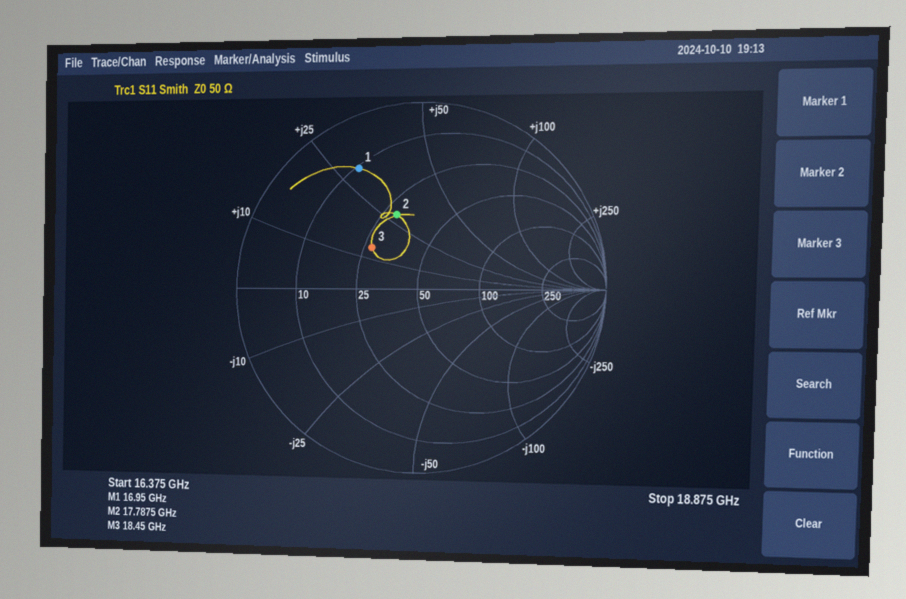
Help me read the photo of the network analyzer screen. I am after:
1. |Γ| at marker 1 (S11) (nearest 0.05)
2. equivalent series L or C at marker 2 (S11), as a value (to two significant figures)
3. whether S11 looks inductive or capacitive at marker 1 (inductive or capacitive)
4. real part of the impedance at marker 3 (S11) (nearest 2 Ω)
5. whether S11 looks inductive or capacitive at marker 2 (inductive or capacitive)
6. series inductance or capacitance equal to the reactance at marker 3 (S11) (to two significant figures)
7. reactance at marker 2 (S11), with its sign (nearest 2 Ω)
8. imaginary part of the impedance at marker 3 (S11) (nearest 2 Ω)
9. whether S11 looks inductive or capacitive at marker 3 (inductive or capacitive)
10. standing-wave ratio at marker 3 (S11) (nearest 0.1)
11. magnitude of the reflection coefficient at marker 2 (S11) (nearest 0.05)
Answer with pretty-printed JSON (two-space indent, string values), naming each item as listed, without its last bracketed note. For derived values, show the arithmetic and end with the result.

{
  "|Γ| at marker 1 (S11)": "0.75",
  "equivalent series L or C at marker 2 (S11), as a value": "L = 28 Ω/(2π × 17.7875 GHz) ≈ 251 pH, so 250 pH to two significant figures",
  "whether S11 looks inductive or capacitive at marker 1": "inductive",
  "real part of the impedance at marker 3 (S11)": "28 Ω",
  "whether S11 looks inductive or capacitive at marker 2": "inductive",
  "series inductance or capacitance equal to the reactance at marker 3 (S11)": "L = 14 Ω/(2π × 18.45 GHz) ≈ 121 pH, so 120 pH to two significant figures",
  "reactance at marker 2 (S11), with its sign": "+28 Ω",
  "imaginary part of the impedance at marker 3 (S11)": "+14 Ω",
  "whether S11 looks inductive or capacitive at marker 3": "inductive",
  "standing-wave ratio at marker 3 (S11)": "2.0",
  "magnitude of the reflection coefficient at marker 2 (S11)": "0.40"
}
